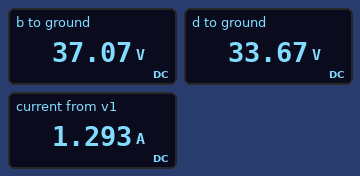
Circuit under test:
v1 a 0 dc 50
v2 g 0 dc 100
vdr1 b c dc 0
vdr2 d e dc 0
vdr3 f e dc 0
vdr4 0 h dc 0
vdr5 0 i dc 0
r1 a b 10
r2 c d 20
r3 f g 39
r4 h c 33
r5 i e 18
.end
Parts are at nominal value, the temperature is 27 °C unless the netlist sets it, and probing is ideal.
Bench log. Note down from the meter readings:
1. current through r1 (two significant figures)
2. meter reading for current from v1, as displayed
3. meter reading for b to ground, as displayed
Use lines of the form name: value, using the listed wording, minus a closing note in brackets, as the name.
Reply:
current through r1: 1.3 A
meter reading for current from v1, as displayed: 1.293 A
meter reading for b to ground, as displayed: 37.07 V
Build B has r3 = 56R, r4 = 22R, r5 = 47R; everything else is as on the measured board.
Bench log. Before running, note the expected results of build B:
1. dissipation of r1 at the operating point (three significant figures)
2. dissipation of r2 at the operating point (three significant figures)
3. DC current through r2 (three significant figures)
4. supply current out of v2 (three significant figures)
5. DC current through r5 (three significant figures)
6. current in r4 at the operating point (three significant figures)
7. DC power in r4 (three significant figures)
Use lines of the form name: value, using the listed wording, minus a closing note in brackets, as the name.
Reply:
dissipation of r1 at the operating point: 20.0 W
dissipation of r2 at the operating point: 922 mW
DC current through r2: 215 mA
supply current out of v2: 1.07 A
DC current through r5: 854 mA
current in r4 at the operating point: 1.63 A
DC power in r4: 58.4 W
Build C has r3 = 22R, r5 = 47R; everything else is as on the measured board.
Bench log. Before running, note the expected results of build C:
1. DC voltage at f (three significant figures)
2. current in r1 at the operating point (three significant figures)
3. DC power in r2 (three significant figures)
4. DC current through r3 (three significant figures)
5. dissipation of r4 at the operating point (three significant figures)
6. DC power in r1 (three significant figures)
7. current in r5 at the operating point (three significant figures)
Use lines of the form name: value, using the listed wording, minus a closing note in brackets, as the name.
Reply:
DC voltage at f: 57.7 V
current in r1 at the operating point: 628 mA
DC power in r2: 9.72 W
DC current through r3: 1.92 A
dissipation of r4 at the operating point: 57.9 W
DC power in r1: 3.94 W
current in r5 at the operating point: 1.23 A
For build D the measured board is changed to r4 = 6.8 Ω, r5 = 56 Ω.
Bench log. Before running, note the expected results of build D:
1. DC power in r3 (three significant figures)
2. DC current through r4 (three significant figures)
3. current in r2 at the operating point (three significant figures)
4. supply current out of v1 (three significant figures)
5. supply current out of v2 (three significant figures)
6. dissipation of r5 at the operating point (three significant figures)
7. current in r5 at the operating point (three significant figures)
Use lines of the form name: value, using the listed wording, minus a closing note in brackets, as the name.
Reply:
DC power in r3: 92.2 W
DC current through r4: 3.47 A
current in r2 at the operating point: 823 mA
supply current out of v1: 2.64 A
supply current out of v2: 1.54 A
dissipation of r5 at the operating point: 28.6 W
current in r5 at the operating point: 715 mA
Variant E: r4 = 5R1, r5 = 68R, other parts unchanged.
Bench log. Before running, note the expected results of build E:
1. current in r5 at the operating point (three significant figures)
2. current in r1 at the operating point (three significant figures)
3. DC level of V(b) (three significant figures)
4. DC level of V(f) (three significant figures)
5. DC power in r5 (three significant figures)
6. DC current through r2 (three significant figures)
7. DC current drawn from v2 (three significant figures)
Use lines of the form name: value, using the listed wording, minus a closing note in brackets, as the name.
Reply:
current in r5 at the operating point: 581 mA
current in r1 at the operating point: 2.98 A
DC level of V(b): 20.2 V
DC level of V(f): 39.5 V
DC power in r5: 23.0 W
DC current through r2: 969 mA
DC current drawn from v2: 1.55 A
